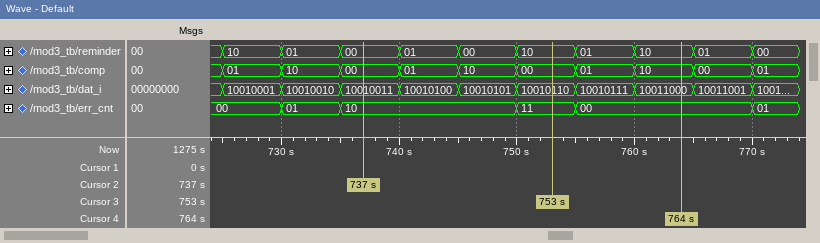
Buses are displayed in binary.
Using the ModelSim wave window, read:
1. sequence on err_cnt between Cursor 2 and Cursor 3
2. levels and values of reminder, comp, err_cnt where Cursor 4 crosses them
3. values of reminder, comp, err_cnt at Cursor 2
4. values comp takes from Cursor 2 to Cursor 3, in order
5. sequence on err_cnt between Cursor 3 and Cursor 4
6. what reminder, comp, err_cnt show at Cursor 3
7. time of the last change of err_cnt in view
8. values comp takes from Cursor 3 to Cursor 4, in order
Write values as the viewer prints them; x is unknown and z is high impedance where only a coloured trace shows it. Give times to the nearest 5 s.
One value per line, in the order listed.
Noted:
10, 11
reminder=10, comp=10, err_cnt=00
reminder=00, comp=00, err_cnt=10
00, 01, 10, 00
11, 00
reminder=10, comp=00, err_cnt=11
770 s
00, 01, 10
